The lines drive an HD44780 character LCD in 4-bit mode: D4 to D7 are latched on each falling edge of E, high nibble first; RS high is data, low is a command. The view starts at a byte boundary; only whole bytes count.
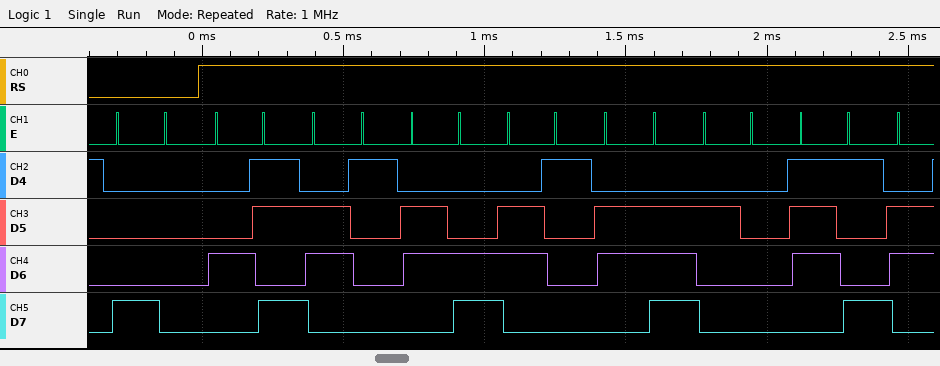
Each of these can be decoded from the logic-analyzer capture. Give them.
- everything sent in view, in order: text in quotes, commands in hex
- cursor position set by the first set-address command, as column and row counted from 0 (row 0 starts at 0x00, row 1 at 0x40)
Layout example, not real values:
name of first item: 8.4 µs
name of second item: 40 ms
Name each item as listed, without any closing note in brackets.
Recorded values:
everything sent in view, in order: text in quotes, commands in hex: 0x80 "Kalan y"
cursor position set by the first set-address command, as column and row counted from 0: column 0, row 0
